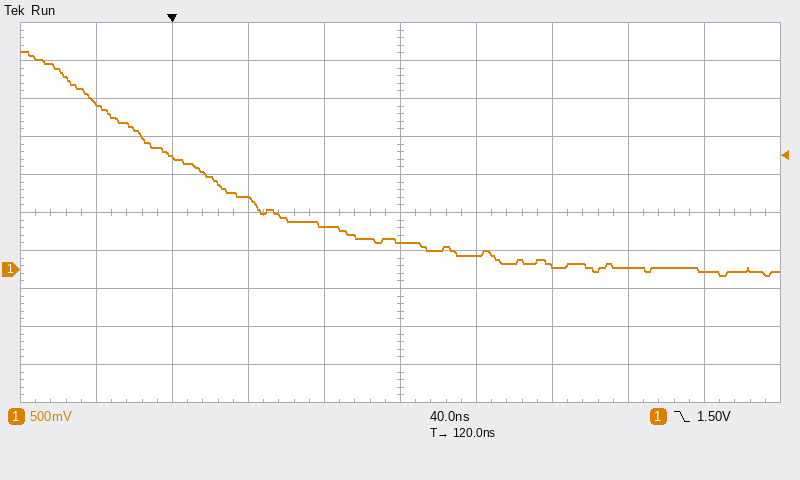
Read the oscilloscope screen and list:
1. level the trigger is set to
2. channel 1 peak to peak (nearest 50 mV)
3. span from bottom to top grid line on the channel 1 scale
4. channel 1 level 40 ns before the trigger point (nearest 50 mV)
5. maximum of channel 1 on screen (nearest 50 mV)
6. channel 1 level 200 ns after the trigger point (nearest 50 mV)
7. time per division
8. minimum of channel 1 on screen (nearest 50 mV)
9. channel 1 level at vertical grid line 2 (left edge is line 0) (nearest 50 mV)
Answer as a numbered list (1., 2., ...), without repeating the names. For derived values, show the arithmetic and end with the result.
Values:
1. 1.50 V
2. 2.85 V − (-100 mV) = 2.95 V
3. 5 V
4. 2.20 V
5. 2.85 V
6. 50 mV
7. 40 ns
8. -100 mV
9. 1.50 V
